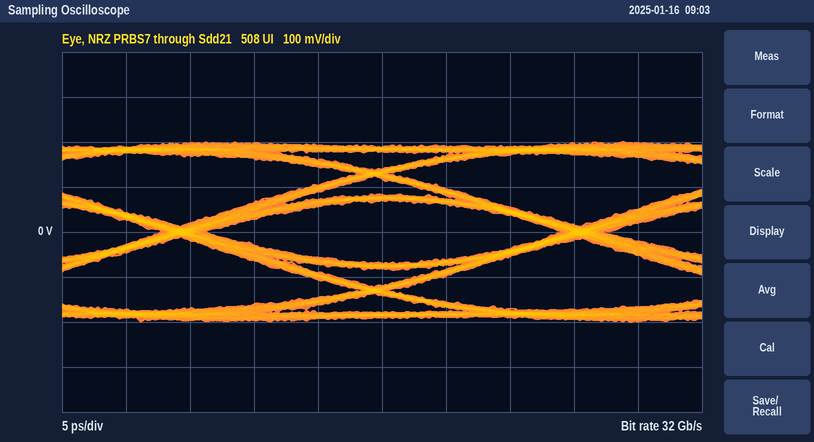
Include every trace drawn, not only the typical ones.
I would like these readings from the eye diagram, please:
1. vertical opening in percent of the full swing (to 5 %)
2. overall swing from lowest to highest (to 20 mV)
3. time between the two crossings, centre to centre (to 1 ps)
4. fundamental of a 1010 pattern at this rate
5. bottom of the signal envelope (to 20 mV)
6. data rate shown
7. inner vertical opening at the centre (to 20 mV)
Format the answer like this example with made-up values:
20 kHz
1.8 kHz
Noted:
35 %
400 mV
31 ps
16 GHz
-200 mV
32 Gb/s
140 mV
